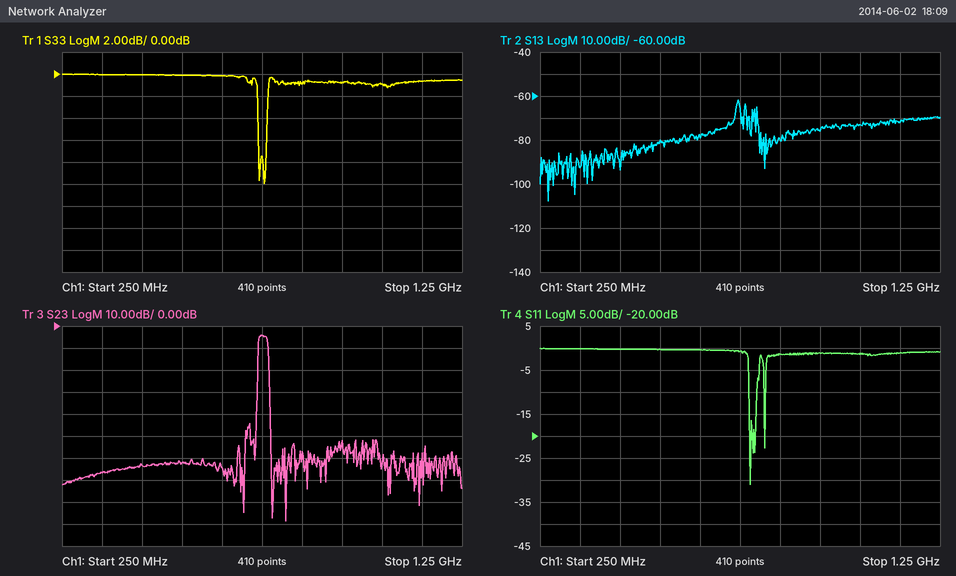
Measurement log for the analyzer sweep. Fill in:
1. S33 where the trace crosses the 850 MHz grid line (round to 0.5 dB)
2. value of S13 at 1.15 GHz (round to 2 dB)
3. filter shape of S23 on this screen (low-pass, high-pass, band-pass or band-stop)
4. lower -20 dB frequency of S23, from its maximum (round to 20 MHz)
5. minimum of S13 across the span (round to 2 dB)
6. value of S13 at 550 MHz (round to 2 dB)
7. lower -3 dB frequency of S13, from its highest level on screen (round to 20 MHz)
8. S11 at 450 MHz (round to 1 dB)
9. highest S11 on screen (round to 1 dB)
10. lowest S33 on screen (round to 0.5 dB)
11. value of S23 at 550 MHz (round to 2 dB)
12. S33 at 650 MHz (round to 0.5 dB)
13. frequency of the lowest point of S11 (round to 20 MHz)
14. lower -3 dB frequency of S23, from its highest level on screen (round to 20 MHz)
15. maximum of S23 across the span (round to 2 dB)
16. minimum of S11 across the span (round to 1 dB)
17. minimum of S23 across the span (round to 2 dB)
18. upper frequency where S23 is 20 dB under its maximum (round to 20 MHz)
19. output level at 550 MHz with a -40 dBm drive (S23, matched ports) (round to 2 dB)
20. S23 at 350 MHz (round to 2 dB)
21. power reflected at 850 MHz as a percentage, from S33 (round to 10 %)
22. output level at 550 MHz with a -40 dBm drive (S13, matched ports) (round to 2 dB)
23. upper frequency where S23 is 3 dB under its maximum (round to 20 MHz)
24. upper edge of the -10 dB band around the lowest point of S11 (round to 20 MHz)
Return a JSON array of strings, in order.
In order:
["-1.0 dB", "-72 dB", "band-pass", "740 MHz", "-108 dB", "-80 dB", "740 MHz", "0 dB", "0 dB", "-10.0 dB", "-62 dB", "0.0 dB", "780 MHz", "740 MHz", "-4 dB", "-31 dB", "-88 dB", "760 MHz", "-102 dBm", "-66 dB", "80 %", "-120 dBm", "760 MHz", "800 MHz"]
